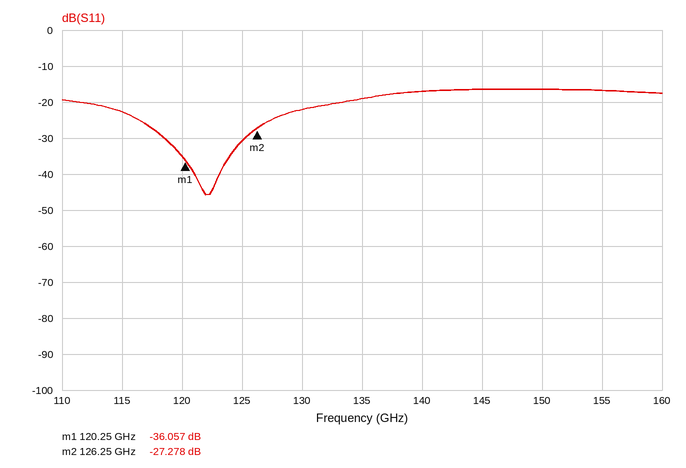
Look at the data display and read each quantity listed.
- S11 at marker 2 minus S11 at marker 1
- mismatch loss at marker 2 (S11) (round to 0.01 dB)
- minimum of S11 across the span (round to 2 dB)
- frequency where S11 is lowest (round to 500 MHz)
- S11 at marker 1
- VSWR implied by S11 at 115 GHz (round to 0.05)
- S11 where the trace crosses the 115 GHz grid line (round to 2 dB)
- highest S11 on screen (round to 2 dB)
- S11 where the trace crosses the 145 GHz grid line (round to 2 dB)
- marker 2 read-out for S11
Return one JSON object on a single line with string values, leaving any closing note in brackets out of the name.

{"S11 at marker 2 minus S11 at marker 1": "8.779 dB", "mismatch loss at marker 2 (S11)": "0.01 dB", "minimum of S11 across the span": "-46 dB", "frequency where S11 is lowest": "122.0 GHz", "S11 at marker 1": "-36.057 dB", "VSWR implied by S11 at 115 GHz": "1.15", "S11 where the trace crosses the 115 GHz grid line": "-22 dB", "highest S11 on screen": "-16 dB", "S11 where the trace crosses the 145 GHz grid line": "-16 dB", "marker 2 read-out for S11": "-27.278 dB"}
